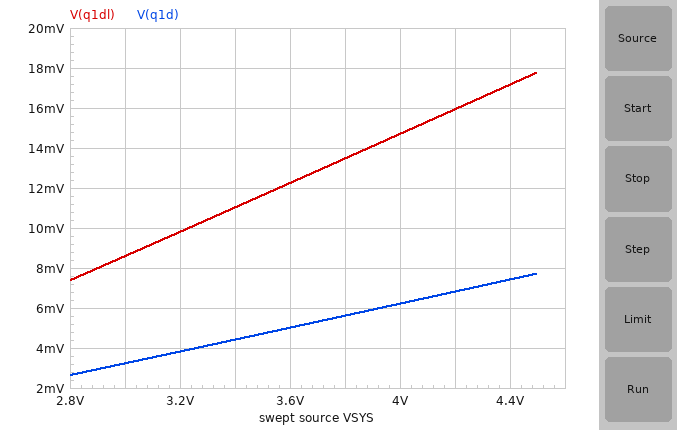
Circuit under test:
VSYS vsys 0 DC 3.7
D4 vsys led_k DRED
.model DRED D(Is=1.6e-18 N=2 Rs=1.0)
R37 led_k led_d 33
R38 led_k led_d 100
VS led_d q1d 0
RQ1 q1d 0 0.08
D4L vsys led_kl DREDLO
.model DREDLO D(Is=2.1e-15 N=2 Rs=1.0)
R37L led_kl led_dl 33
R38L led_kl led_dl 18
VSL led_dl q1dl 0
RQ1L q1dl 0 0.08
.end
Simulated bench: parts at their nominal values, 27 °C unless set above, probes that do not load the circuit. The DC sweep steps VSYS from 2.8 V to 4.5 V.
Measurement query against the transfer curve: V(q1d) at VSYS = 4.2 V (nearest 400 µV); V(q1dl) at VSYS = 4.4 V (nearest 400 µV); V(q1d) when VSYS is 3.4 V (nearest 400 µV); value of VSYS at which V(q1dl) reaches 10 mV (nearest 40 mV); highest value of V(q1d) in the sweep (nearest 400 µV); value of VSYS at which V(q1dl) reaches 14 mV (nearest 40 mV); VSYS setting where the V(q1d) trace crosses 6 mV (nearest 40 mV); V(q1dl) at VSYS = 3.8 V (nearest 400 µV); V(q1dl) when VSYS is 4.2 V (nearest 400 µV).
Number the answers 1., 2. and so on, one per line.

1. 6.8 mV
2. 17.2 mV
3. 4.4 mV
4. 3.24 V
5. 7.6 mV
6. 3.88 V
7. 3.92 V
8. 13.6 mV
9. 16.0 mV
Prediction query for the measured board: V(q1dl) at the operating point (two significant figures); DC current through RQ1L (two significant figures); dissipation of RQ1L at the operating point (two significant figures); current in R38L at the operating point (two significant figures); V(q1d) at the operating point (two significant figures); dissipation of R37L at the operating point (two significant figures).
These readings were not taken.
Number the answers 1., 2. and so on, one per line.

1. 13 mV
2. 160 mA
3. 2.1 mW
4. 100 mA
5. 5.3 mV
6. 110 mW
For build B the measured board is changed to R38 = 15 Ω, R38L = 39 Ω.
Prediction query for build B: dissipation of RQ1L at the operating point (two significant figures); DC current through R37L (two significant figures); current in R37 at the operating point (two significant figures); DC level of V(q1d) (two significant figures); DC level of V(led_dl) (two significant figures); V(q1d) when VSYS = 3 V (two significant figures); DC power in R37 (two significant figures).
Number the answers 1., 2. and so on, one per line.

1. 950 µW
2. 59 mA
3. 46 mA
4. 12 mV
5. 8.7 mV
6. 7.1 mV
7. 70 mW
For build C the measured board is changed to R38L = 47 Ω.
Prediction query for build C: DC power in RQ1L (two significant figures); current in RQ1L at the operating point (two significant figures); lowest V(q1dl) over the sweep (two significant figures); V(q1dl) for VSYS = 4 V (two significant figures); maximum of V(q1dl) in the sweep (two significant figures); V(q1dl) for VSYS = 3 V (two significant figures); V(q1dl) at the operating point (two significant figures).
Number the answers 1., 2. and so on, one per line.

1. 820 µW
2. 100 mA
3. 4.7 mV
4. 9.2 mV
5. 11 mV
6. 5.4 mV
7. 8.1 mV
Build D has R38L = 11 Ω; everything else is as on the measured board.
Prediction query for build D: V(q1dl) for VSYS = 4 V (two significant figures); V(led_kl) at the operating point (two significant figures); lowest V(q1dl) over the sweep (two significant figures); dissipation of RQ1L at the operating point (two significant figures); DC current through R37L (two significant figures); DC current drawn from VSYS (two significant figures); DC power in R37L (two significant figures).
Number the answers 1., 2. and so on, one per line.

1. 20 mV
2. 1.8 V
3. 9.9 mV
4. 3.8 mW
5. 54 mA
6. 280 mA
7. 98 mW
